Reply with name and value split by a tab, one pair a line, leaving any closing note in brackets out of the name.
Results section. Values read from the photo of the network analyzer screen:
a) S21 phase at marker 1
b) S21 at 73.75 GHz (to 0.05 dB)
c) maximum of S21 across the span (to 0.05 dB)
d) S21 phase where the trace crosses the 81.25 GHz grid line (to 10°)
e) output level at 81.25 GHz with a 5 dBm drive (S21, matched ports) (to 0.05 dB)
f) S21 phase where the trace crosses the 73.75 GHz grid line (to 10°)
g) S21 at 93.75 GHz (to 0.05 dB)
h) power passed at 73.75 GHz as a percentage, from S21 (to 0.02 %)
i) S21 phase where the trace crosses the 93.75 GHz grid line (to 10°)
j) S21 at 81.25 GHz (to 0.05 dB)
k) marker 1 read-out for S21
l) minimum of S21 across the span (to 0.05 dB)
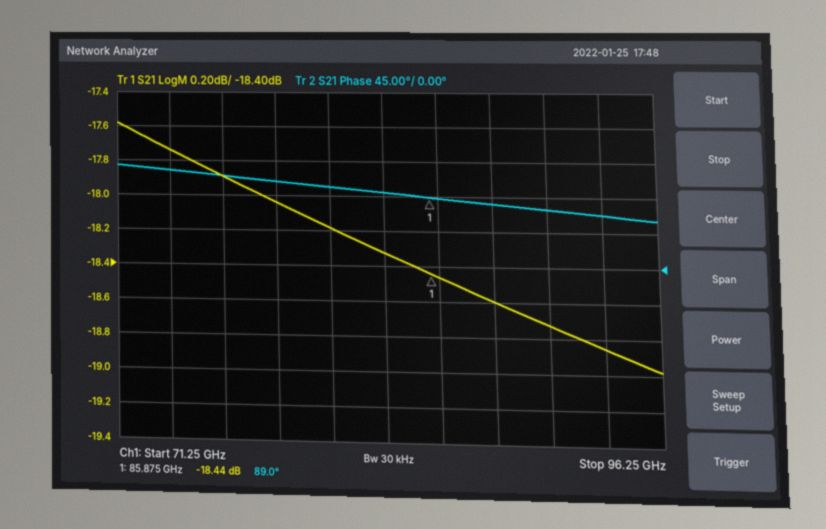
S21 phase at marker 1	89.0°
S21 at 73.75 GHz	-17.75 dB
maximum of S21 across the span	-17.60 dB
S21 phase where the trace crosses the 81.25 GHz grid line	100°
output level at 81.25 GHz with a 5 dBm drive (S21, matched ports)	-13.20 dBm
S21 phase where the trace crosses the 73.75 GHz grid line	120°
S21 at 93.75 GHz	-18.85 dB
power passed at 73.75 GHz as a percentage, from S21	1.68 %
S21 phase where the trace crosses the 93.75 GHz grid line	70°
S21 at 81.25 GHz	-18.20 dB
marker 1 read-out for S21	-18.44 dB
minimum of S21 across the span	-19.00 dB
